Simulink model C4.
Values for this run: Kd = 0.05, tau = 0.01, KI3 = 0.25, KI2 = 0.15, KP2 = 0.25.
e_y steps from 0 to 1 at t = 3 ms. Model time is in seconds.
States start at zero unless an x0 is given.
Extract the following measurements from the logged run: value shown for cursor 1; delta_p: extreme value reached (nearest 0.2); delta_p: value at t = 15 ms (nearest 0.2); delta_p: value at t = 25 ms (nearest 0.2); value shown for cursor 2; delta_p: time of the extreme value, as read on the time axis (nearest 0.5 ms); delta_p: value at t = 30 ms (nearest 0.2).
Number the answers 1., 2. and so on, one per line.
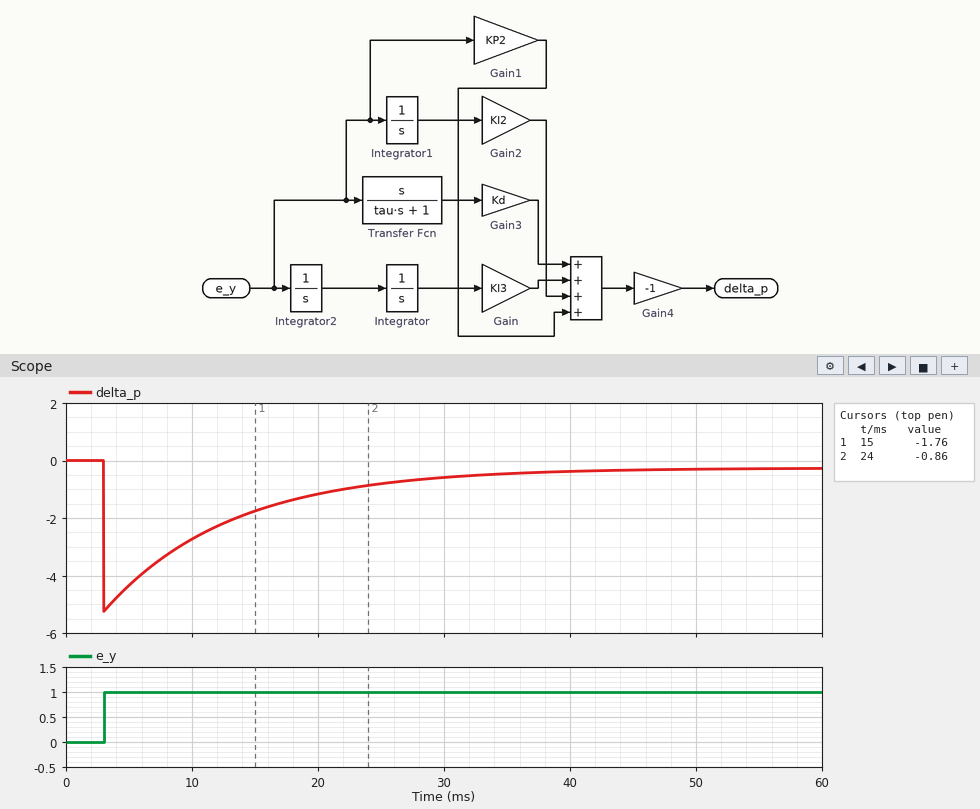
1. -1.76
2. -5.2
3. -1.8
4. -0.8
5. -0.86
6. 3.0 ms
7. -0.6
